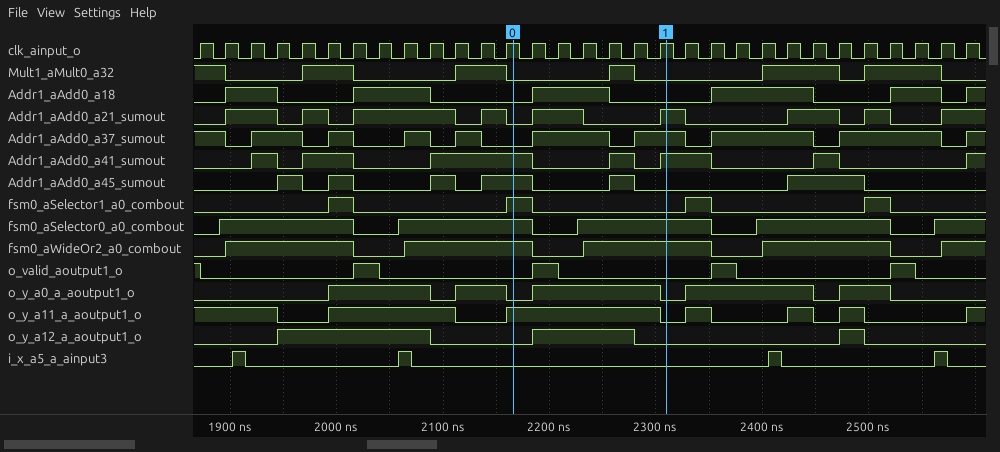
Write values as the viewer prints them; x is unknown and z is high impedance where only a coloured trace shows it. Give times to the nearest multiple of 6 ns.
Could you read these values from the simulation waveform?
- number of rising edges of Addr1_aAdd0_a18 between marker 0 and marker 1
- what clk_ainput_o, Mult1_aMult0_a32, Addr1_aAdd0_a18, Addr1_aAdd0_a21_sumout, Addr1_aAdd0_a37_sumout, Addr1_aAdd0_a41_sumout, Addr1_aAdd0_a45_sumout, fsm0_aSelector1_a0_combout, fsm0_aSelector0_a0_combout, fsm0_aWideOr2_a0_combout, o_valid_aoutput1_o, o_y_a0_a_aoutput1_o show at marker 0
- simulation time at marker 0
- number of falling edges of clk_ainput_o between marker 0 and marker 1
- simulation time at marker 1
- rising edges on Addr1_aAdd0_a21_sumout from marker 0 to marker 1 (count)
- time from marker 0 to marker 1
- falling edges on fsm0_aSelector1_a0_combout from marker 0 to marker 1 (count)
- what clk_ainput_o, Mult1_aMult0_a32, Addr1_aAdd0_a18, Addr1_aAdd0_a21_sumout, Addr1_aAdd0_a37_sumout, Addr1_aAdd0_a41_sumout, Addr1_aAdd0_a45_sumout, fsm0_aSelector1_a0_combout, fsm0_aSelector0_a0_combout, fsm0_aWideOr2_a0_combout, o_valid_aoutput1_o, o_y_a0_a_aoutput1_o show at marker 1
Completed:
1
clk_ainput_o=1, Mult1_aMult0_a32=0, Addr1_aAdd0_a18=0, Addr1_aAdd0_a21_sumout=0, Addr1_aAdd0_a37_sumout=0, Addr1_aAdd0_a41_sumout=1, Addr1_aAdd0_a45_sumout=1, fsm0_aSelector1_a0_combout=1, fsm0_aSelector0_a0_combout=1, fsm0_aWideOr2_a0_combout=1, o_valid_aoutput1_o=0, o_y_a0_a_aoutput1_o=0
2166 ns
6
2310 ns
2
144 ns
1
clk_ainput_o=1, Mult1_aMult0_a32=0, Addr1_aAdd0_a18=0, Addr1_aAdd0_a21_sumout=1, Addr1_aAdd0_a37_sumout=1, Addr1_aAdd0_a41_sumout=1, Addr1_aAdd0_a45_sumout=0, fsm0_aSelector1_a0_combout=0, fsm0_aSelector0_a0_combout=1, fsm0_aWideOr2_a0_combout=1, o_valid_aoutput1_o=0, o_y_a0_a_aoutput1_o=0
